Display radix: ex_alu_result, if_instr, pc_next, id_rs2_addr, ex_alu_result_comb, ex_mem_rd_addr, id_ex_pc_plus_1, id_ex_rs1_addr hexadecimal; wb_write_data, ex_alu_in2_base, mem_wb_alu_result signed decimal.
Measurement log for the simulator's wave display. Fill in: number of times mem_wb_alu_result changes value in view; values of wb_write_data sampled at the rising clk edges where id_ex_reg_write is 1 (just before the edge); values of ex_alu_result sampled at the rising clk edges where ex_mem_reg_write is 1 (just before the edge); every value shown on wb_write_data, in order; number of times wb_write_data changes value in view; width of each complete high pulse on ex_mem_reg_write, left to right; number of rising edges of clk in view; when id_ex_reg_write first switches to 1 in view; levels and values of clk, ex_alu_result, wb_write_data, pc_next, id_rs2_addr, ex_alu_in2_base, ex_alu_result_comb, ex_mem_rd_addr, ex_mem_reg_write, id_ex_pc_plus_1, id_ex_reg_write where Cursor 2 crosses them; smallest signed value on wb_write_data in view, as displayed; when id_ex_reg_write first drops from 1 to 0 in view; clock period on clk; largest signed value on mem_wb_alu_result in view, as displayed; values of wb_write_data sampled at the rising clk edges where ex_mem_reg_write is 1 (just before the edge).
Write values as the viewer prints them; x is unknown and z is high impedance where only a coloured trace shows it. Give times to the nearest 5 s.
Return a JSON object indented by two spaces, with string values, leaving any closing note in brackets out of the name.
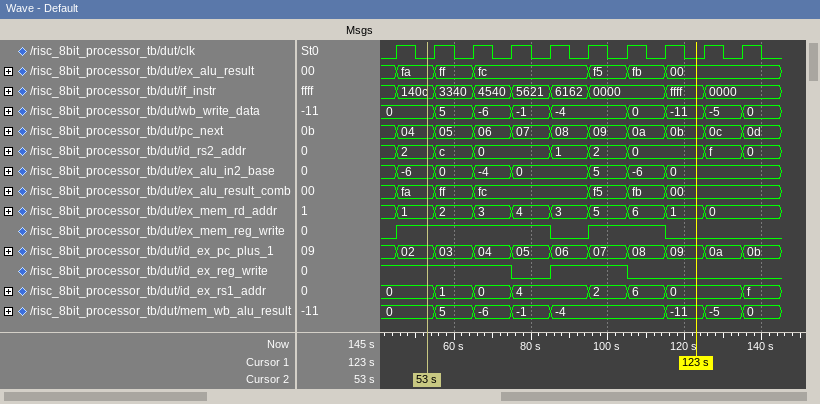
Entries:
{
  "number of times mem_wb_alu_result changes value in view": "7",
  "values of wb_write_data sampled at the rising clk edges where id_ex_reg_write is 1": "0, 0, 5, -6, -4, -4",
  "values of ex_alu_result sampled at the rising clk edges where ex_mem_reg_write is 1": "fa, ff, fc, fc, f5, fb",
  "every value shown on wb_write_data, in order": "0, 5, -6, -1, -4, 0, -11, -5, 0",
  "number of times wb_write_data changes value in view": "8",
  "width of each complete high pulse on ex_mem_reg_write, left to right": "40 s, 20 s",
  "number of rising edges of clk in view": "10",
  "when id_ex_reg_write first switches to 1 in view": "85 s",
  "levels and values of clk, ex_alu_result, wb_write_data, pc_next, id_rs2_addr, ex_alu_in2_base, ex_alu_result_comb, ex_mem_rd_addr, ex_mem_reg_write, id_ex_pc_plus_1, id_ex_reg_write where Cursor 2 crosses them": "clk=0, ex_alu_result=fa, wb_write_data=0, pc_next=04, id_rs2_addr=2, ex_alu_in2_base=-6, ex_alu_result_comb=fa, ex_mem_rd_addr=1, ex_mem_reg_write=1, id_ex_pc_plus_1=02, id_ex_reg_write=1",
  "smallest signed value on wb_write_data in view, as displayed": "-11",
  "when id_ex_reg_write first drops from 1 to 0 in view": "75 s",
  "clock period on clk": "10 s",
  "largest signed value on mem_wb_alu_result in view, as displayed": "5",
  "values of wb_write_data sampled at the rising clk edges where ex_mem_reg_write is 1": "0, 5, -6, -1, -4, 0"
}
